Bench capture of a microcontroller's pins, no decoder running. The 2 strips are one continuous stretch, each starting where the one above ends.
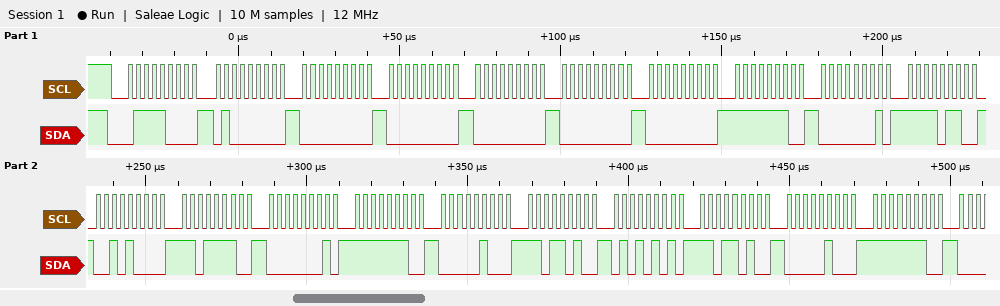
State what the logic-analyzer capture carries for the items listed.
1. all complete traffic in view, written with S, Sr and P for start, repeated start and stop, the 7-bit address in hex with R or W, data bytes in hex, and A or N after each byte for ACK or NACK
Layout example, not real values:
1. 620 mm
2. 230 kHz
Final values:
1. S 3CW A 40 A 00 A 00 A 00 A 00 A 00 A FE A 01 A F6 A 28 A DE A 01 A FE A 04 A DA A 55 A DA A 04 A FE A
